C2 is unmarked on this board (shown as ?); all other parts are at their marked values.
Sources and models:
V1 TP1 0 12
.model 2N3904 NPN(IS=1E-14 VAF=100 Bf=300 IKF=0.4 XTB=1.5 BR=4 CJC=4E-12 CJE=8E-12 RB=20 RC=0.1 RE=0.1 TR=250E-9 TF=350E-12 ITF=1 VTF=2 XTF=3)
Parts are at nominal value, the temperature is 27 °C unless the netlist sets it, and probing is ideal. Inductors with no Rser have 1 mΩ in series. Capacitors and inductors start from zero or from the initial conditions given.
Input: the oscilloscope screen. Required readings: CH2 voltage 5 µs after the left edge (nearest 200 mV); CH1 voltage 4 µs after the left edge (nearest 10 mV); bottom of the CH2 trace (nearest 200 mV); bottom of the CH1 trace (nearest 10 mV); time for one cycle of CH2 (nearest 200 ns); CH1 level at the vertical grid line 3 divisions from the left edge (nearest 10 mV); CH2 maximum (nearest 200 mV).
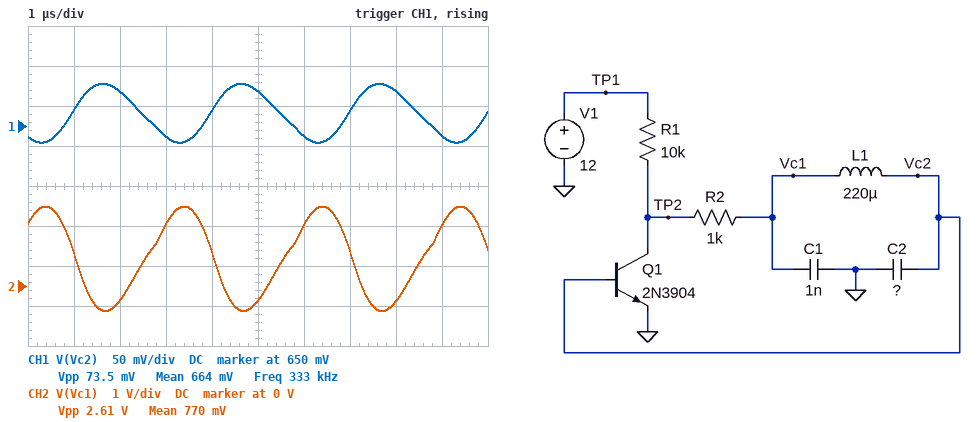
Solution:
-400 mV
670 mV
-600 mV
630 mV
3.0 µs
640 mV
2.0 V
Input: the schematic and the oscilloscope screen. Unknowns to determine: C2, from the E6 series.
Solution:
33 nF
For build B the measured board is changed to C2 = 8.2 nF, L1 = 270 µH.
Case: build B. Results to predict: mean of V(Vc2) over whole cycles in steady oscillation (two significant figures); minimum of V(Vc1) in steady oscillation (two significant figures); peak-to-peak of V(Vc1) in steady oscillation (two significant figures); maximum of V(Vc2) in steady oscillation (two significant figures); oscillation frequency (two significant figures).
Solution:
640 mV
-980 mV
3.3 V
770 mV
320 kHz
